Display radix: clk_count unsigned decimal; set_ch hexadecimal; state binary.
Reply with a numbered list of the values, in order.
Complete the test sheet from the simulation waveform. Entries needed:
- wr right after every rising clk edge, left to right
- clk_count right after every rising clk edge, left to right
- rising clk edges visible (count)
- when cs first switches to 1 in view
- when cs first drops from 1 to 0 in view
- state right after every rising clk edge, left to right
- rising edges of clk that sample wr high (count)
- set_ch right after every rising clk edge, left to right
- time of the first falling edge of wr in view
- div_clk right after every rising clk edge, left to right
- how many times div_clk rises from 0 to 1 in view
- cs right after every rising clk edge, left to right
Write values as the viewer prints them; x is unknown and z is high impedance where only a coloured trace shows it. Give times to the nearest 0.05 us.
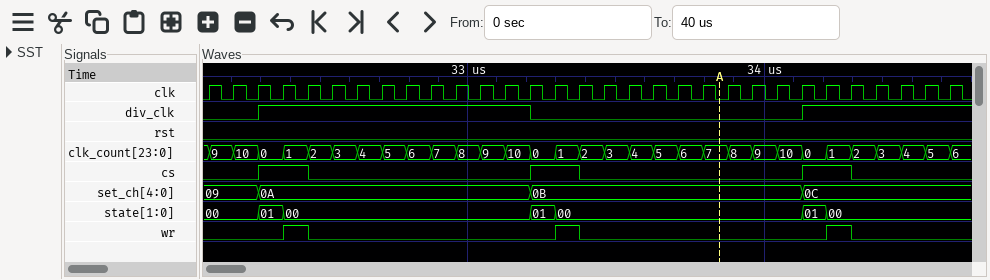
1. 0 0 0 1 0 0 0 0 0 0 0 0 0 0 1 0 0 0 0 0 0 0 0 0 0 1 0 0 0 0 0
2. 9, 10, 0, 1, 2, 3, 4, 5, 6, 7, 8, 9, 10, 0, 1, 2, 3, 4, 5, 6, 7, 8, 9, 10, 0, 1, 2, 3, 4, 5, 6
3. 31
4. 32.3 us
5. 32.45 us
6. 00, 00, 01, 00, 00, 00, 00, 00, 00, 00, 00, 00, 00, 01, 00, 00, 00, 00, 00, 00, 00, 00, 00, 00, 01, 00, 00, 00, 00, 00, 00
7. 3
8. 09, 09, 0A, 0A, 0A, 0A, 0A, 0A, 0A, 0A, 0A, 0A, 0A, 0B, 0B, 0B, 0B, 0B, 0B, 0B, 0B, 0B, 0B, 0B, 0C, 0C, 0C, 0C, 0C, 0C, 0C
9. 32.45 us
10. 0 0 1 1 1 1 1 1 1 1 1 1 1 0 0 0 0 0 0 0 0 0 0 0 1 1 1 1 1 1 1
11. 2
12. 0 0 1 1 0 0 0 0 0 0 0 0 0 1 1 0 0 0 0 0 0 0 0 0 1 1 0 0 0 0 0
